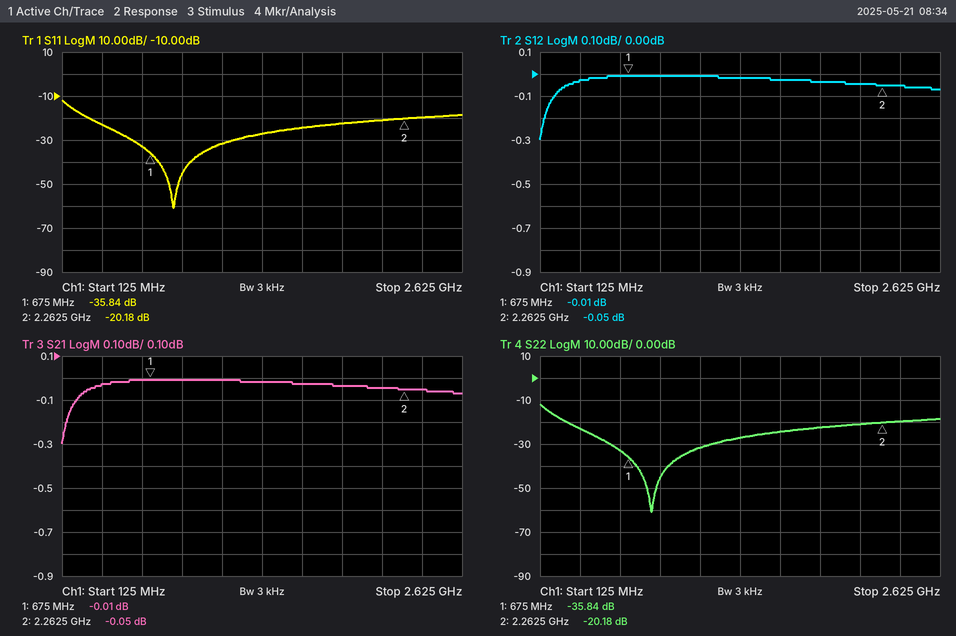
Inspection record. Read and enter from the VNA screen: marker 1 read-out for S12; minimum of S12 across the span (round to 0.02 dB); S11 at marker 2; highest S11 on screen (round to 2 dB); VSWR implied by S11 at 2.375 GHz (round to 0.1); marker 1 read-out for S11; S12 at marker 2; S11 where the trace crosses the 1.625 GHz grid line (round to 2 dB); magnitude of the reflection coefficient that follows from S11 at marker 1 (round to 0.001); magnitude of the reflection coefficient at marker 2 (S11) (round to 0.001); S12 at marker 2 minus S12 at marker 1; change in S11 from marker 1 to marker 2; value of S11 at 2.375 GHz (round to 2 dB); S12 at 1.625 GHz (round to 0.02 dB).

-0.01 dB
-0.30 dB
-20.18 dB
-12 dB
1.2
-35.84 dB
-0.05 dB
-24 dB
0.016
0.098
-0.04 dB
15.66 dB
-20 dB
-0.02 dB
